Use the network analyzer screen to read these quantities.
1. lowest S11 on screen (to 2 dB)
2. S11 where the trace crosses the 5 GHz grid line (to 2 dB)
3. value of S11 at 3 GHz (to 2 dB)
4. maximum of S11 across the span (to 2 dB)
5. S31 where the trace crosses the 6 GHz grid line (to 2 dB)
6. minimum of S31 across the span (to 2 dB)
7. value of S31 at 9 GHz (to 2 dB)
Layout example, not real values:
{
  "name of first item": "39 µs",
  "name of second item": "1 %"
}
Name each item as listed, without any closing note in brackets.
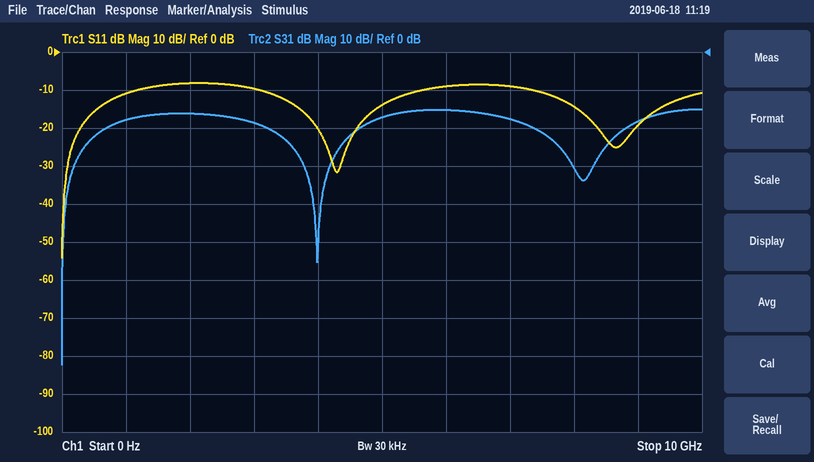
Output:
{
  "lowest S11 on screen": "-54 dB",
  "S11 where the trace crosses the 5 GHz grid line": "-14 dB",
  "value of S11 at 3 GHz": "-10 dB",
  "maximum of S11 across the span": "-8 dB",
  "S31 where the trace crosses the 6 GHz grid line": "-16 dB",
  "minimum of S31 across the span": "-82 dB",
  "value of S31 at 9 GHz": "-18 dB"
}
